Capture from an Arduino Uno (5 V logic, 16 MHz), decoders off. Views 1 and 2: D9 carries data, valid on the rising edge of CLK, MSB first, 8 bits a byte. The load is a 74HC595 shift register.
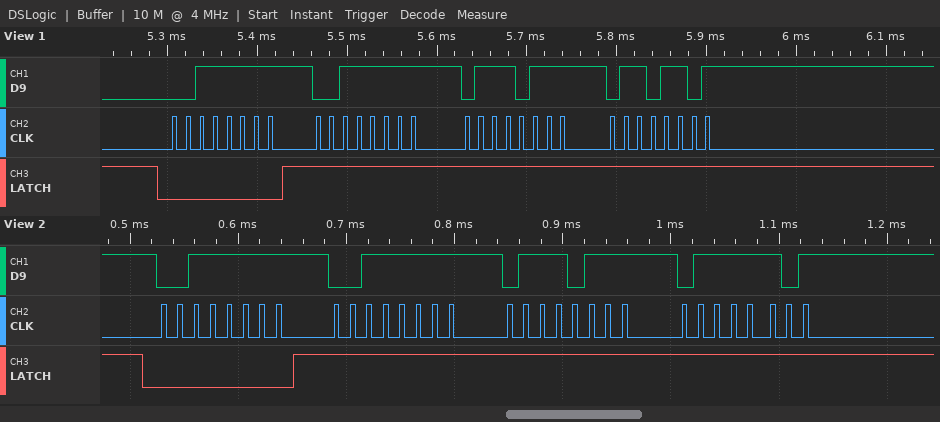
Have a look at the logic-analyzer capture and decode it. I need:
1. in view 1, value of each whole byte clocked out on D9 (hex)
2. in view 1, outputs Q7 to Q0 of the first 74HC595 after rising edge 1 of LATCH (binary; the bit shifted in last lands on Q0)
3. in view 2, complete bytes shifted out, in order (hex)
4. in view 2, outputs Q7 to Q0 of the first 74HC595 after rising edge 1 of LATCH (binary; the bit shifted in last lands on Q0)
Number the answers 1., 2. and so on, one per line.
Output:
1. 3F 3F 77 6D
2. 00111111
3. 3F 3F 77 7D
4. 00111111
